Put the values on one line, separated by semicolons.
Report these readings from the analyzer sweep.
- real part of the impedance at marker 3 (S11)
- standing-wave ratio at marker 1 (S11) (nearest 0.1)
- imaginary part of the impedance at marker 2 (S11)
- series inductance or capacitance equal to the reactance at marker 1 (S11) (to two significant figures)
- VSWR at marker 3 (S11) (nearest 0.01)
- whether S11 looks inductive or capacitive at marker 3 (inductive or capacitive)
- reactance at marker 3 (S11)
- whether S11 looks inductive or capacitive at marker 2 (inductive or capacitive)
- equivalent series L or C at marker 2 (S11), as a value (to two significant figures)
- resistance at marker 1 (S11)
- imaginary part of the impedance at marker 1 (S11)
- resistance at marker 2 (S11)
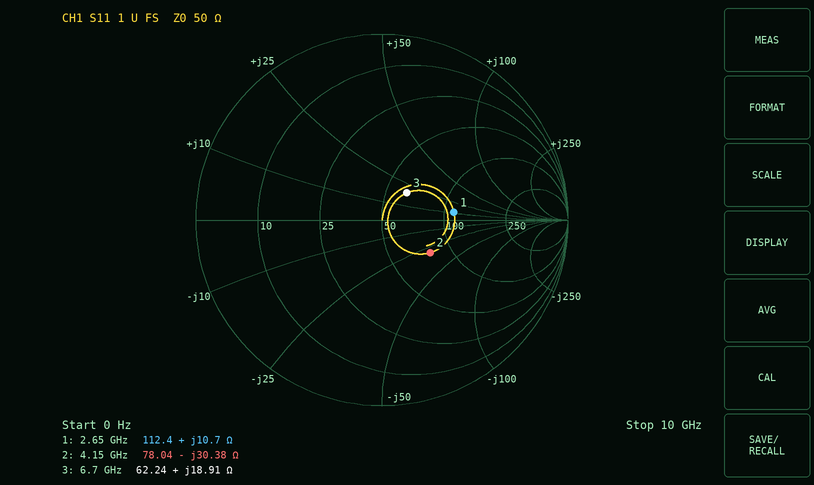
62.24 Ω; 2.3; -30.38 Ω; 640 pH; 1.49; inductive; +18.91 Ω; capacitive; 1.3 pF; 112.4 Ω; +10.7 Ω; 78.04 Ω
